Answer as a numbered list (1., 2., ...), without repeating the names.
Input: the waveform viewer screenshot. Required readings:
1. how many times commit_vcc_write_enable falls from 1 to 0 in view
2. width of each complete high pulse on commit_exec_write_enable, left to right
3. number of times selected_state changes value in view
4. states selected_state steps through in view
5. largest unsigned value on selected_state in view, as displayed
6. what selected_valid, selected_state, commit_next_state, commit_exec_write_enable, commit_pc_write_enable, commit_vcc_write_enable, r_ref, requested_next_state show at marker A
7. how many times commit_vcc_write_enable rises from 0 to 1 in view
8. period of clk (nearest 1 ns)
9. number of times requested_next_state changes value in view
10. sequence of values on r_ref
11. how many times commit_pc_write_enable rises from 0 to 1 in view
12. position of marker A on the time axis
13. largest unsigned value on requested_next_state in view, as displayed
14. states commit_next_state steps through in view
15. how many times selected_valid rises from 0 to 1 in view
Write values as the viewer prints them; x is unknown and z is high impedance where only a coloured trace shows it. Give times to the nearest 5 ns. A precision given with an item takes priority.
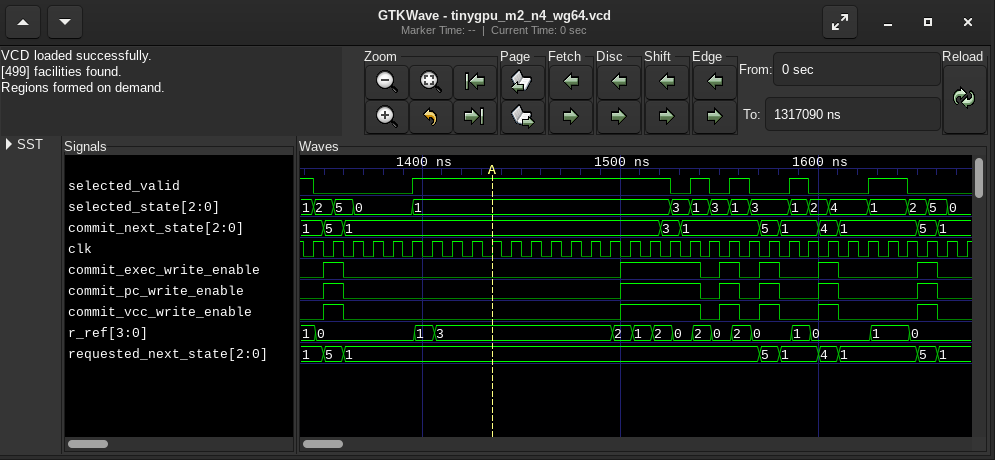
1. 6
2. 10 ns, 40 ns, 10 ns, 10 ns, 10 ns, 10 ns
3. 16
4. 1, 2, 5, 0, 1, 3, 1, 3, 1, 3, 1, 2, 4, 1, 2, 5, 0
5. 5
6. selected_valid=1, selected_state=1, commit_next_state=1, commit_exec_write_enable=0, commit_pc_write_enable=0, commit_vcc_write_enable=0, r_ref=3, requested_next_state=1
7. 6
8. 10 ns
9. 8
10. 1, 0, 1, 3, 2, 1, 2, 0, 2, 0, 2, 0, 1, 0, 1, 0
11. 6
12. 1435 ns
13. 5
14. 1, 5, 1, 3, 1, 5, 1, 4, 1, 5, 1
15. 5
